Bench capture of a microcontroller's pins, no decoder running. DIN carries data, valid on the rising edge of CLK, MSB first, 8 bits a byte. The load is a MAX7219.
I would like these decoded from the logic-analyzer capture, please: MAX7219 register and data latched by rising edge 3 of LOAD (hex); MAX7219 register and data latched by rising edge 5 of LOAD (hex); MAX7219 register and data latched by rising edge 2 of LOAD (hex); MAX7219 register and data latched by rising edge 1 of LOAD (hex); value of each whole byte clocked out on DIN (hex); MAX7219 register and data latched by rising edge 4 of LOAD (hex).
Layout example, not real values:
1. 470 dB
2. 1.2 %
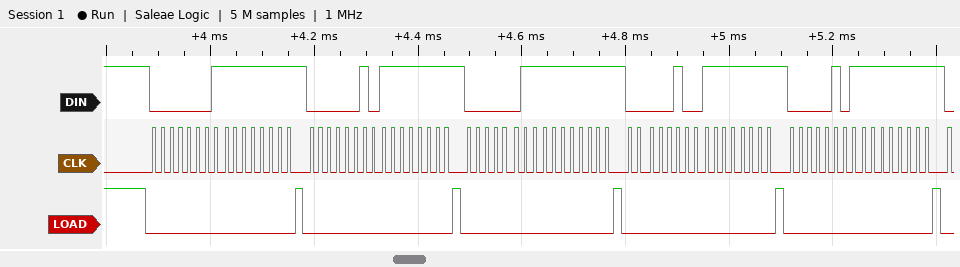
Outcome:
1. register 0x3, data 0xFF
2. register 0x5, data 0xFF
3. register 0x2, data 0xFF
4. register 0x1, data 0xFF
5. 01 FF 02 FF 03 FF 04 FF 05 FF
6. register 0x4, data 0xFF
